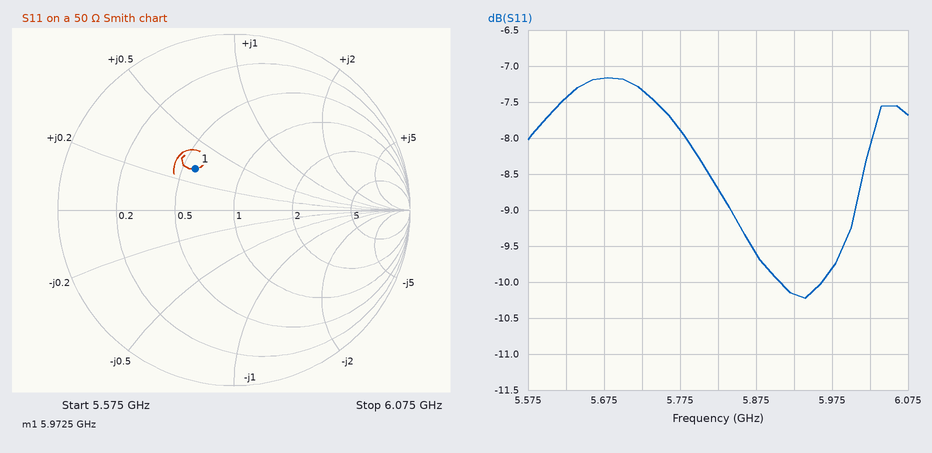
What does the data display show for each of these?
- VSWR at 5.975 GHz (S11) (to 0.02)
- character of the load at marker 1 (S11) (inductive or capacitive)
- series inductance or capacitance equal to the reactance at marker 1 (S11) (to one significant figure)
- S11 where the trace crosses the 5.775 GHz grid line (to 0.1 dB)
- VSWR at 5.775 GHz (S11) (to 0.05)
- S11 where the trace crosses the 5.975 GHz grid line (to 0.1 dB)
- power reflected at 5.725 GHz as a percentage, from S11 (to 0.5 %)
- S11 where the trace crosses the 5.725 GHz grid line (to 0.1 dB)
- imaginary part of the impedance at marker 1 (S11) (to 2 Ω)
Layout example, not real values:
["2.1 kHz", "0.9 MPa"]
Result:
["1.96", "inductive", "400 pH", "-7.9 dB", "2.35", "-9.8 dB", "18.5 %", "-7.3 dB", "+16 Ω"]
